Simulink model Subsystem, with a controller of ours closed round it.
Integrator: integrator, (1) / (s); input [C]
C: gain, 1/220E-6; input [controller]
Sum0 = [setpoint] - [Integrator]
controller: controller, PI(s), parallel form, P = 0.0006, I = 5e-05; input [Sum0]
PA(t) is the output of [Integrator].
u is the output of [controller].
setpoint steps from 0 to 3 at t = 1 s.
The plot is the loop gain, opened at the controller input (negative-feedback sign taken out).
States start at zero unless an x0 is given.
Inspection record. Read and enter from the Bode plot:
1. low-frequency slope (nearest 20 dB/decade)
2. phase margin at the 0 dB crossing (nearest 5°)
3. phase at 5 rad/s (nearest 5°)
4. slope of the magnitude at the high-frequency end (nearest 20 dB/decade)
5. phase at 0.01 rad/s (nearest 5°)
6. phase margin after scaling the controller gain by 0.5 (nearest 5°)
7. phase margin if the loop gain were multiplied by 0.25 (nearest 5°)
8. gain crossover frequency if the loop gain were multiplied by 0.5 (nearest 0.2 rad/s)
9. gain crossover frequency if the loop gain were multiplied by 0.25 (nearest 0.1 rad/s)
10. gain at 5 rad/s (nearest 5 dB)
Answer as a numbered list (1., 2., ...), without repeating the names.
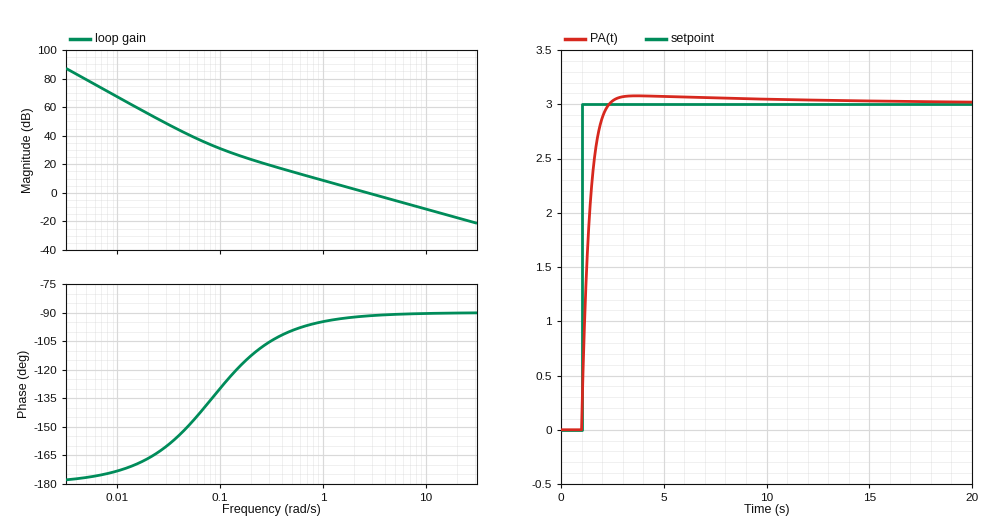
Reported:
1. -40 dB/decade
2. 90°
3. -90°
4. -20 dB/decade
5. -175°
6. 85°
7. 85°
8. 1.4 rad/s
9. 0.7 rad/s
10. -5 dB
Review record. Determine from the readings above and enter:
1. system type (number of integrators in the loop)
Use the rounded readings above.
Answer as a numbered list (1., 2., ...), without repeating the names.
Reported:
1. 2
